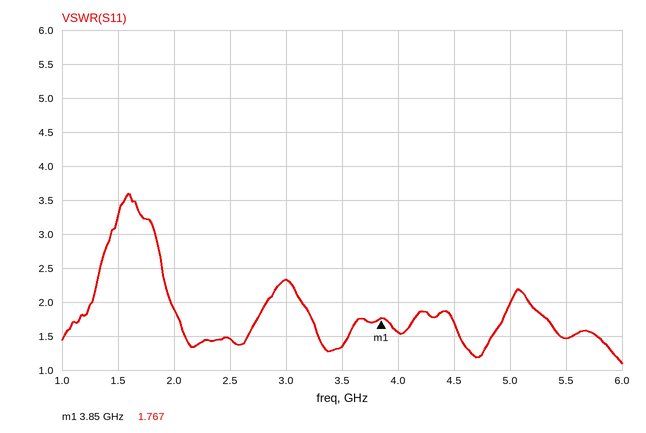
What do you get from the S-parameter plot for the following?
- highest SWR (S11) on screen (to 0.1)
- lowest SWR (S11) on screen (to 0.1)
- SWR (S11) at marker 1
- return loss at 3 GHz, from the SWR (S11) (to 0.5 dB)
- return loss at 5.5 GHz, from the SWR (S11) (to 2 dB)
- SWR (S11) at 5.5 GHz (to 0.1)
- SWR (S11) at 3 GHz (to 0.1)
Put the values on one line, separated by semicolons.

3.6; 1.1; 1.767; 8.0 dB; 14 dB; 1.5; 2.3
